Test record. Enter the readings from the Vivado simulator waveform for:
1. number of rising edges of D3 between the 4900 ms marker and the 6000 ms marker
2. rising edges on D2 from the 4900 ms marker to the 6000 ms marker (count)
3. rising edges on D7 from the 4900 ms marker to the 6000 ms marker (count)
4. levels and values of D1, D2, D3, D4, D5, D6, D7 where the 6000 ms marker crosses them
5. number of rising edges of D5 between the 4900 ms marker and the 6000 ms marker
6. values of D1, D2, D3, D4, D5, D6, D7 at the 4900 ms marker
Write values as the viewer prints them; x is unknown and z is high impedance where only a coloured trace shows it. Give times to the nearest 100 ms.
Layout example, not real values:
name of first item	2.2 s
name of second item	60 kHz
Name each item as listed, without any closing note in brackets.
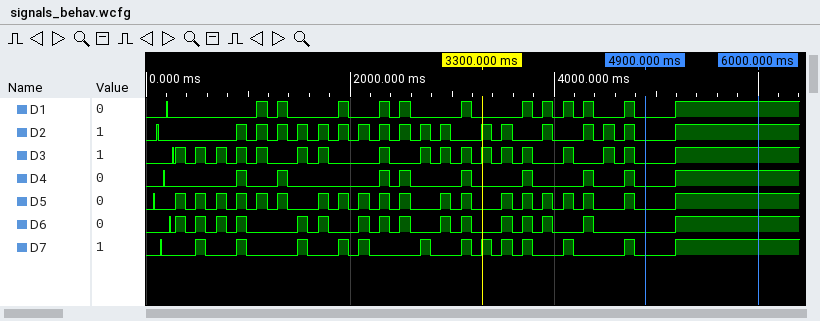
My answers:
number of rising edges of D3 between the 4900 ms marker and the 6000 ms marker	1
rising edges on D2 from the 4900 ms marker to the 6000 ms marker	1
rising edges on D7 from the 4900 ms marker to the 6000 ms marker	1
levels and values of D1, D2, D3, D4, D5, D6, D7 where the 6000 ms marker crosses them	D1=1, D2=1, D3=1, D4=1, D5=1, D6=1, D7=1
number of rising edges of D5 between the 4900 ms marker and the 6000 ms marker	1
values of D1, D2, D3, D4, D5, D6, D7 at the 4900 ms marker	D1=0, D2=0, D3=0, D4=0, D5=0, D6=0, D7=0
